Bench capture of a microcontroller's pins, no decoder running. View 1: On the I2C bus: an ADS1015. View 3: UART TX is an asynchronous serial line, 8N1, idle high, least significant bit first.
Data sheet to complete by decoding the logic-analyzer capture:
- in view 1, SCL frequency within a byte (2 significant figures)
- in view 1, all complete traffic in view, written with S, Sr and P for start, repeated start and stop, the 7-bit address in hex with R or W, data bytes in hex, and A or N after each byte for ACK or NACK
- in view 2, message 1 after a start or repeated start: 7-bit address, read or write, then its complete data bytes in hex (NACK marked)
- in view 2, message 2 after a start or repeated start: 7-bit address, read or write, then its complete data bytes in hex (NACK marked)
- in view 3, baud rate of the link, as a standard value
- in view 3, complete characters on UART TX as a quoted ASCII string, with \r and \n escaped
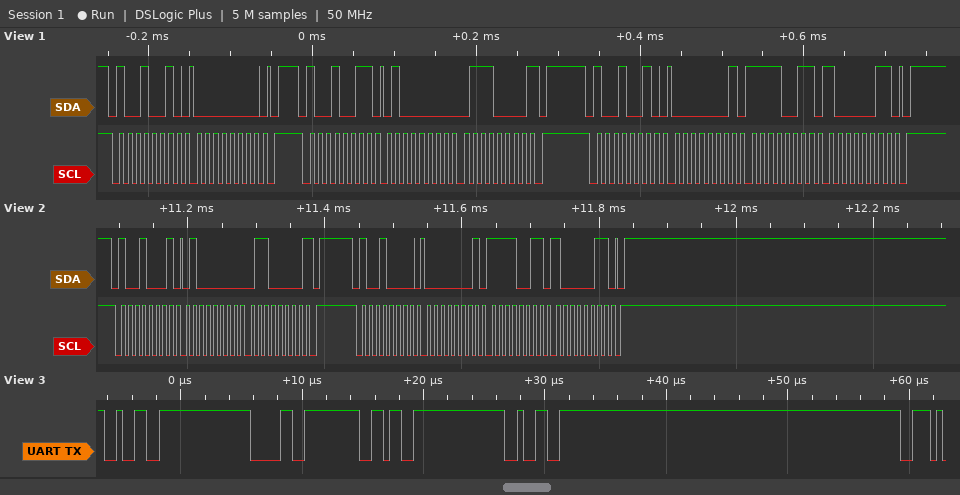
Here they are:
100 kHz
S 49W A 00 A P S 49R A 40 A 70 N P S 49W A 01 A F3 A 83 A P
0x48 read: 40 60 NACK
0x48 write: 01 F3 83
2000000 baud
"2062"
